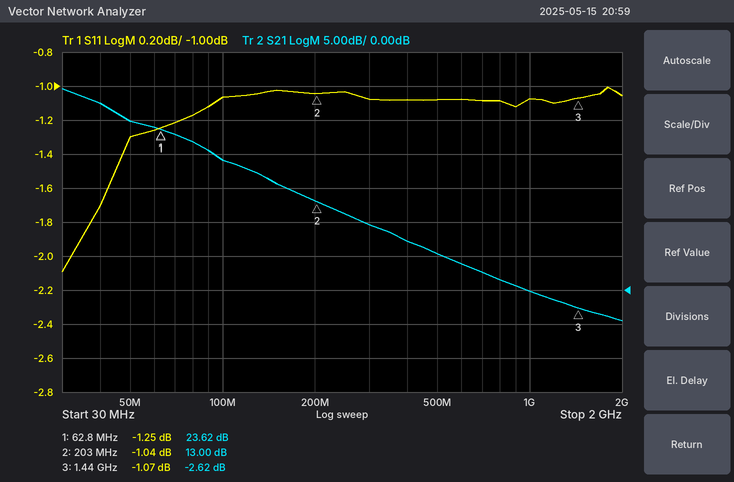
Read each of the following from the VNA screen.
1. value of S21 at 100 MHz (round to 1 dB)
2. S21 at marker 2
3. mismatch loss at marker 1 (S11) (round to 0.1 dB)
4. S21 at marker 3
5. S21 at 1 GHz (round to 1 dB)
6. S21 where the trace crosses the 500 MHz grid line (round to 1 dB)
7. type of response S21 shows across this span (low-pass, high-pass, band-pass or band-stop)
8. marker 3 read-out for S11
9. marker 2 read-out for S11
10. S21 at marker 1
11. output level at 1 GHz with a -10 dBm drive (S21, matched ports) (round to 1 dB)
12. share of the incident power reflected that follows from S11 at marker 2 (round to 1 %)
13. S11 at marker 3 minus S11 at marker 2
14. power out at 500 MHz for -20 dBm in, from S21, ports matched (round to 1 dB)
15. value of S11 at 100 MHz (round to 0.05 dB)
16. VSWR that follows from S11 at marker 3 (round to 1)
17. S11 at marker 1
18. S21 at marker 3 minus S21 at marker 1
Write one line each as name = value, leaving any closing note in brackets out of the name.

value of S21 at 100 MHz = 19 dB
S21 at marker 2 = 13.00 dB
mismatch loss at marker 1 (S11) = 6.0 dB
S21 at marker 3 = -2.62 dB
S21 at 1 GHz = 0 dB
S21 where the trace crosses the 500 MHz grid line = 5 dB
type of response S21 shows across this span = low-pass
marker 3 read-out for S11 = -1.07 dB
marker 2 read-out for S11 = -1.04 dB
S21 at marker 1 = 23.62 dB
output level at 1 GHz with a -10 dBm drive (S21, matched ports) = -10 dBm
share of the incident power reflected that follows from S11 at marker 2 = 79 %
S11 at marker 3 minus S11 at marker 2 = -0.03 dB
power out at 500 MHz for -20 dBm in, from S21, ports matched = -15 dBm
value of S11 at 100 MHz = -1.05 dB
VSWR that follows from S11 at marker 3 = 16
S11 at marker 1 = -1.25 dB
S21 at marker 3 minus S21 at marker 1 = -26.24 dB
